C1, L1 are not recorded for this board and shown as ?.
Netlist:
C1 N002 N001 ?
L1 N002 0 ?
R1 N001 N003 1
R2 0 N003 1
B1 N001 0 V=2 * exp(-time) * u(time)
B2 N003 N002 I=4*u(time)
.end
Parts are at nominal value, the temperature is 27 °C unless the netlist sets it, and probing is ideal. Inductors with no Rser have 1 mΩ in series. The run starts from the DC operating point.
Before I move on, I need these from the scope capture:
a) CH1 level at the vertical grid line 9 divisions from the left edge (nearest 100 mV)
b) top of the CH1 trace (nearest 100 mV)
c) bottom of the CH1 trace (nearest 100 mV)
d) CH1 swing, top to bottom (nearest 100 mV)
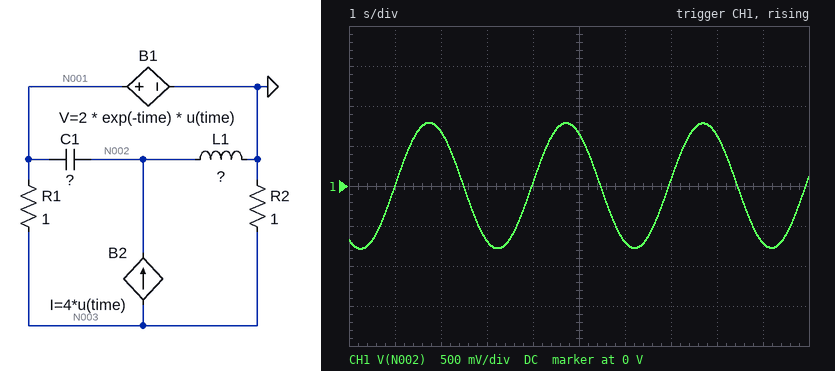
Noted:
-700 mV
800 mV
-800 mV
1.6 V
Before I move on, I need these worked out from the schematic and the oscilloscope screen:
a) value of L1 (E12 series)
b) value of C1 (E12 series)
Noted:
330 mH
680 mF
